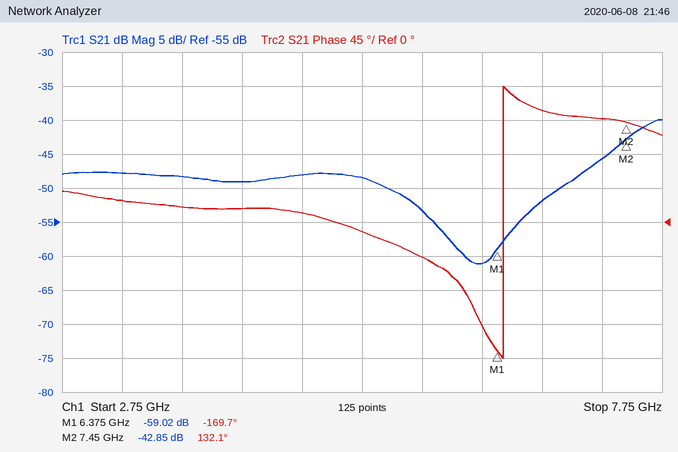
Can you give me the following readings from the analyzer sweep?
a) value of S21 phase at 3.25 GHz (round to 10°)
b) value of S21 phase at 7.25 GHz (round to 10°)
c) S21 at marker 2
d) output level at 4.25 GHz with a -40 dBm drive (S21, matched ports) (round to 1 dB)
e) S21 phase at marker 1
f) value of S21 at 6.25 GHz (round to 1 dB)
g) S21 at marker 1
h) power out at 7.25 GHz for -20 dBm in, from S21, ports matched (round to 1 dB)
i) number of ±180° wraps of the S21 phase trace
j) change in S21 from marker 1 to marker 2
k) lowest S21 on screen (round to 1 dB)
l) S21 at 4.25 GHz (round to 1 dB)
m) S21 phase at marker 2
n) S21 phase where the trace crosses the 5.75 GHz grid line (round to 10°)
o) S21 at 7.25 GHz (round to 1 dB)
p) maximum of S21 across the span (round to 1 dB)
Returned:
30°
140°
-42.85 dB
-89 dBm
-169.7°
-61 dB
-59.02 dB
-66 dBm
1
16.17 dB
-61 dB
-49 dB
132.1°
-50°
-46 dB
-40 dB
